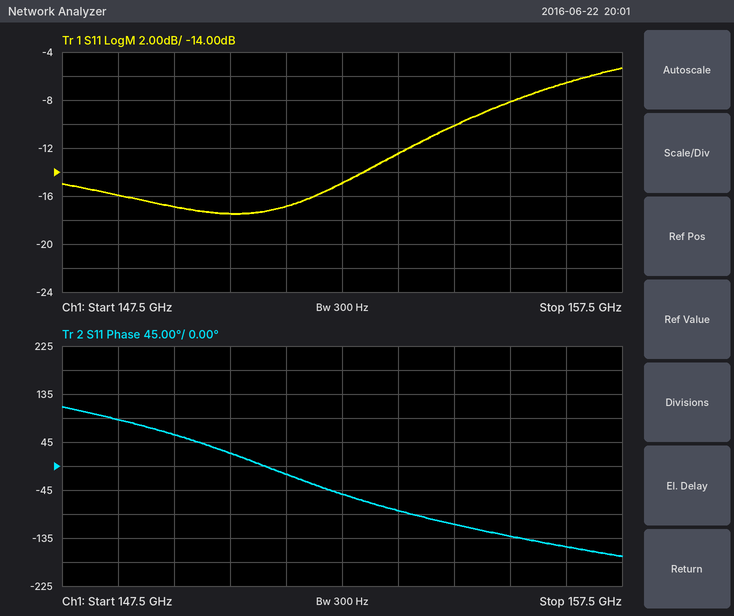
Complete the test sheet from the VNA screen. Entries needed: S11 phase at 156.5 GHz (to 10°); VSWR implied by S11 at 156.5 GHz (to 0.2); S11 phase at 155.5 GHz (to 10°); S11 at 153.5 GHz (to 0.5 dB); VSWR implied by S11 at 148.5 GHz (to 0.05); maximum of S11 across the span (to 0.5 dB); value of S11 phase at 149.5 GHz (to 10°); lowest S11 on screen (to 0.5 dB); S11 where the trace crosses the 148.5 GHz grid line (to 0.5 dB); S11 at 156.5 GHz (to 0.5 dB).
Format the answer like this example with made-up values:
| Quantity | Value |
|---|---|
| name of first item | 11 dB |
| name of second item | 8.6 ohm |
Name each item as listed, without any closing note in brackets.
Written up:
| Quantity | Value |
|---|---|
| S11 phase at 156.5 GHz | -150° |
| VSWR implied by S11 at 156.5 GHz | 2.8 |
| S11 phase at 155.5 GHz | -130° |
| S11 at 153.5 GHz | -12.5 dB |
| VSWR implied by S11 at 148.5 GHz | 1.40 |
| maximum of S11 across the span | -5.5 dB |
| value of S11 phase at 149.5 GHz | 60° |
| lowest S11 on screen | -17.5 dB |
| S11 where the trace crosses the 148.5 GHz grid line | -16.0 dB |
| S11 at 156.5 GHz | -6.5 dB |
